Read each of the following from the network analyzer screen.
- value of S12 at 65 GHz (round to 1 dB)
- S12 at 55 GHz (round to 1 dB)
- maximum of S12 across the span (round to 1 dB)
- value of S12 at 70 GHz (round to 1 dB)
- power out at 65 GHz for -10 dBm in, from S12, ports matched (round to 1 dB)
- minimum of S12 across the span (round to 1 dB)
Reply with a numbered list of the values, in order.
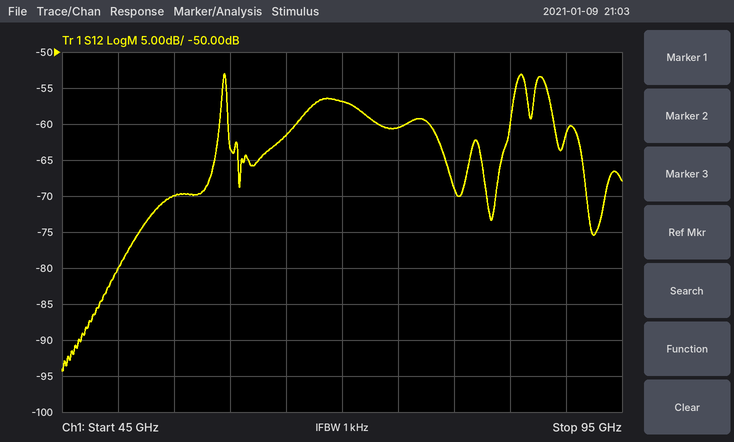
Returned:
1. -62 dB
2. -70 dB
3. -53 dB
4. -57 dB
5. -72 dBm
6. -94 dB
